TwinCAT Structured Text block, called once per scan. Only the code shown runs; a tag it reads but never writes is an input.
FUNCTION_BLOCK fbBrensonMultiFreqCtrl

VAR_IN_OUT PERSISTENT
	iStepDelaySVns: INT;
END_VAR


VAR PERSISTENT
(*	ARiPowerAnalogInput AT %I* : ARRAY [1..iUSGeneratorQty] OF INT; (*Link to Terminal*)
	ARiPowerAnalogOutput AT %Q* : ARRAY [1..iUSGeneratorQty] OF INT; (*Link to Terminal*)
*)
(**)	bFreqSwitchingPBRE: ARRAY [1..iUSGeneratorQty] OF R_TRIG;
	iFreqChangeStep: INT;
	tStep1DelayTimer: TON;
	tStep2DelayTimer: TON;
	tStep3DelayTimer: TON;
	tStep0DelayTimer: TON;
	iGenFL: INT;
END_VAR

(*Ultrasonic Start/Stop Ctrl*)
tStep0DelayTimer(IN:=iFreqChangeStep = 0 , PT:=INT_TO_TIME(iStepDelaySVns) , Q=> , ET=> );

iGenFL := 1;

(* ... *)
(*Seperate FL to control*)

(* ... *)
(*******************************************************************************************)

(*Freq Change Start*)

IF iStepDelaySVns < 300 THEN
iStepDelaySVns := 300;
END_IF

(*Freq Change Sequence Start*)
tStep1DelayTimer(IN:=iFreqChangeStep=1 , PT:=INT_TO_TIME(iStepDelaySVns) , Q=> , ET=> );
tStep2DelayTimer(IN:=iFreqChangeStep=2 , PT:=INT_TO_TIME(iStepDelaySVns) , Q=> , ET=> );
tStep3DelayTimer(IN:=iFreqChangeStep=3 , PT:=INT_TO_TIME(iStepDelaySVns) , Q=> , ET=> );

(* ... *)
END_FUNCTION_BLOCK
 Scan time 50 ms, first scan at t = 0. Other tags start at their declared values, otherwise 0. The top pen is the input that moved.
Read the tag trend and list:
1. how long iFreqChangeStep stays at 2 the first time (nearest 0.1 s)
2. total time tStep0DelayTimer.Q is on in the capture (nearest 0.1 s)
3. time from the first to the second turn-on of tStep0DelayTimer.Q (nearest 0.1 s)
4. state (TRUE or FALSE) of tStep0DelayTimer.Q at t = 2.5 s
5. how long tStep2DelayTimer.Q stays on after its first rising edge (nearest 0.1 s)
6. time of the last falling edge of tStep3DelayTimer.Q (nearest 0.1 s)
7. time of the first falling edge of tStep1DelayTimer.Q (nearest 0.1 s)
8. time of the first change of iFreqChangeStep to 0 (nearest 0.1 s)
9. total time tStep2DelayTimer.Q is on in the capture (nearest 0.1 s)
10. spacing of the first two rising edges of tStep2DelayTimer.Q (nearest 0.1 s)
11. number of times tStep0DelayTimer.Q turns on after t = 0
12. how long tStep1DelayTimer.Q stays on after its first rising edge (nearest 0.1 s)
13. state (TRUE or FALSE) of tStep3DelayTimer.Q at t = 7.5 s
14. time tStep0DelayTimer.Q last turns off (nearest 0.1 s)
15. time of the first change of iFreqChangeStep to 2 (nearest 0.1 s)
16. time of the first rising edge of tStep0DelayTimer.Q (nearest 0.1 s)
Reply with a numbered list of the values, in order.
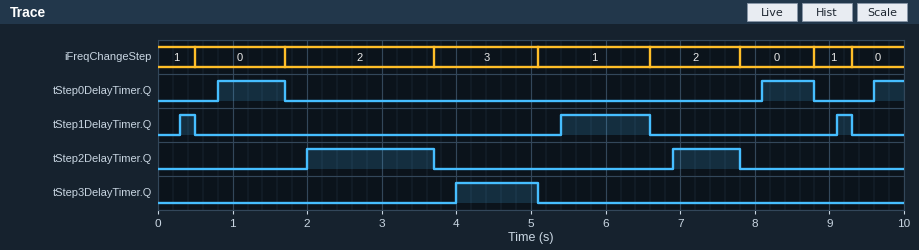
1. 2.0 s
2. 2.0 s
3. 7.3 s
4. FALSE
5. 1.7 s
6. 5.1 s
7. 0.5 s
8. 0.5 s
9. 2.6 s
10. 4.9 s
11. 3
12. 0.2 s
13. FALSE
14. 8.8 s
15. 1.7 s
16. 0.8 s
